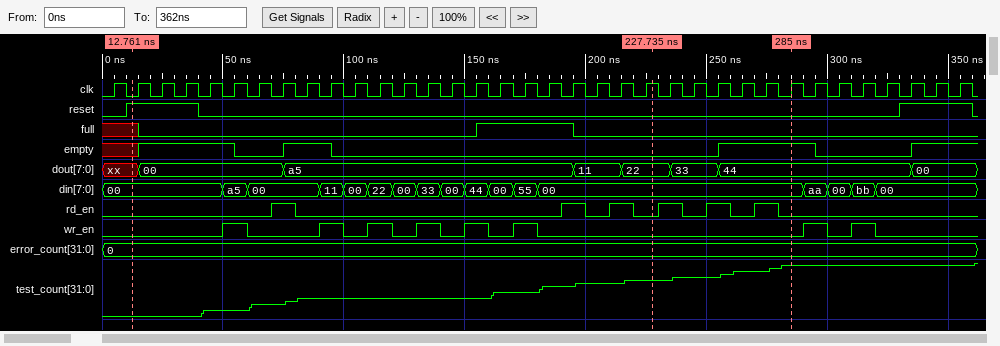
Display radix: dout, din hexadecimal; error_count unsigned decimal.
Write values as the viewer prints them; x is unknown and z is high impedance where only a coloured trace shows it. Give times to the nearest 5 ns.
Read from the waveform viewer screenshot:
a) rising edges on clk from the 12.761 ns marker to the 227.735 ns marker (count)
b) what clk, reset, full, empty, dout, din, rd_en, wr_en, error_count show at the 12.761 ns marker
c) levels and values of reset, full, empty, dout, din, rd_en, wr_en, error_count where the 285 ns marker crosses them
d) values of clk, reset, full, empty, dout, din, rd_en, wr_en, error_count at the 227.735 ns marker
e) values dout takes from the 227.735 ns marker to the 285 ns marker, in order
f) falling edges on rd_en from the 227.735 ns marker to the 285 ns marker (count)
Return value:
22
clk=0, reset=1, full=x, empty=x, dout=xx, din=00, rd_en=0, wr_en=0, error_count=0
reset=0, full=0, empty=1, dout=44, din=00, rd_en=0, wr_en=0, error_count=0
clk=1, reset=0, full=0, empty=0, dout=22, din=00, rd_en=0, wr_en=0, error_count=0
22, 33, 44
3
